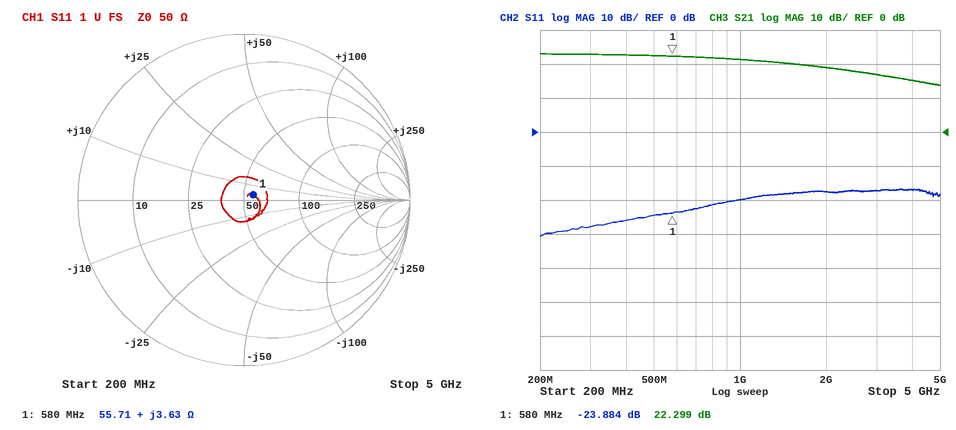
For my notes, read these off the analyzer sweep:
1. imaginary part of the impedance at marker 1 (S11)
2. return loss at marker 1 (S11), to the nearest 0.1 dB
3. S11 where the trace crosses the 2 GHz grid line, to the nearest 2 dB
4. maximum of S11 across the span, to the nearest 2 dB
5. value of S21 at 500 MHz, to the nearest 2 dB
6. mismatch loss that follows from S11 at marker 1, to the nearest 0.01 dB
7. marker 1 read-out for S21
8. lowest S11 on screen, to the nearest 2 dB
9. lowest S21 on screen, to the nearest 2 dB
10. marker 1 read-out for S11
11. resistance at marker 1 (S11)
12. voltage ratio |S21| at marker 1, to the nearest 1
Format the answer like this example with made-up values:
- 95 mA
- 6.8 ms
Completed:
- +3.63 Ω
- 23.9 dB
- -18 dB
- -16 dB
- 22 dB
- 0.02 dB
- 22.299 dB
- -30 dB
- 14 dB
- -23.884 dB
- 55.71 Ω
- 13
